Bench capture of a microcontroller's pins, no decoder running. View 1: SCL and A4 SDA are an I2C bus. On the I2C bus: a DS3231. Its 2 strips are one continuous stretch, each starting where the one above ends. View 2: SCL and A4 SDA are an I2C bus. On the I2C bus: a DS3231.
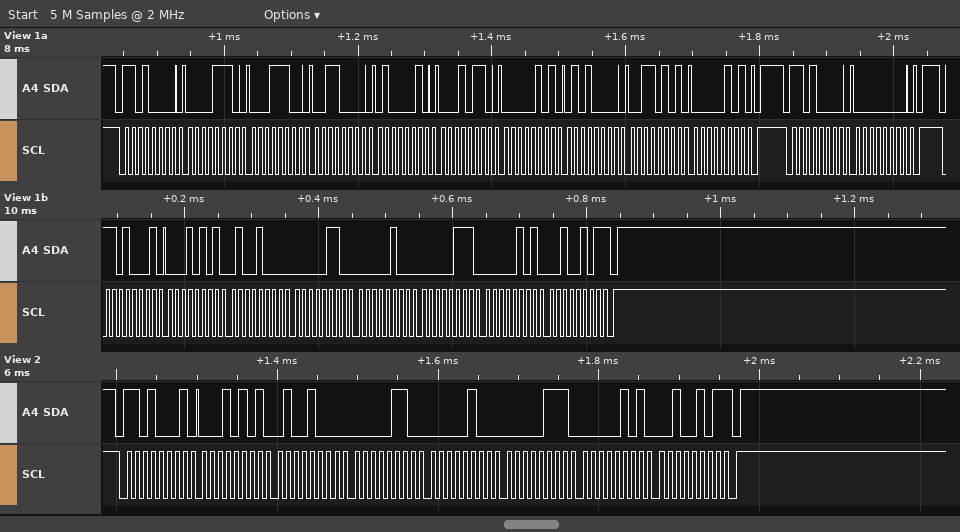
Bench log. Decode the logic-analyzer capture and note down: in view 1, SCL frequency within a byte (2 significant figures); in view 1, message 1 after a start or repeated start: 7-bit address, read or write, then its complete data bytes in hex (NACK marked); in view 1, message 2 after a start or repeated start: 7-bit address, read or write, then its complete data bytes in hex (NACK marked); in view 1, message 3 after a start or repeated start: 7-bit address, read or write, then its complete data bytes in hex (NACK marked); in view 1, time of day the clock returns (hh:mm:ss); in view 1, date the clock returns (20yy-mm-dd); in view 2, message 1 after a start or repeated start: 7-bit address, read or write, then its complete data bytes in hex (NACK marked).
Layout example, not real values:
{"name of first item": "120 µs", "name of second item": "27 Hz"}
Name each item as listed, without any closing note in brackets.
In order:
{"in view 1, SCL frequency within a byte": "100 kHz", "in view 1, message 1 after a start or repeated start: 7-bit address, read or write, then its complete data bytes in hex": "0x68 write: 0E 1C 30 42 16 05 50 35 05", "in view 1, message 2 after a start or repeated start: 7-bit address, read or write, then its complete data bytes in hex": "0x68 write: 00", "in view 1, message 3 after a start or repeated start: 7-bit address, read or write, then its complete data bytes in hex": "0x68 read: 15 48 06 04 07 05 25 NACK", "in view 1, time of day the clock returns": "06:48:15", "in view 1, date the clock returns": "2025-05-07", "in view 2, message 1 after a start or repeated start: 7-bit address, read or write, then its complete data bytes in hex": "0x68 read: 15 48 06 04 07 05 25 NACK"}
